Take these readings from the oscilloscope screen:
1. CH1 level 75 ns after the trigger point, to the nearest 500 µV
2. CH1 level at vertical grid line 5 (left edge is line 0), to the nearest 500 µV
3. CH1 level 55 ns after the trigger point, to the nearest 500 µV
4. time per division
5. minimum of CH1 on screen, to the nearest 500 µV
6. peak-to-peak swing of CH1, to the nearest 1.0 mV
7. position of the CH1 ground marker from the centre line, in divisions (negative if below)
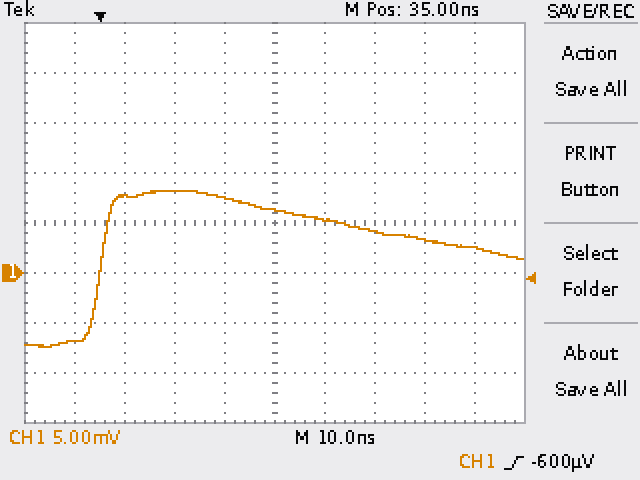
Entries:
2.5 mV
6.5 mV
4.0 mV
10 ns
-7.5 mV
16.0 mV
-1.0 div
